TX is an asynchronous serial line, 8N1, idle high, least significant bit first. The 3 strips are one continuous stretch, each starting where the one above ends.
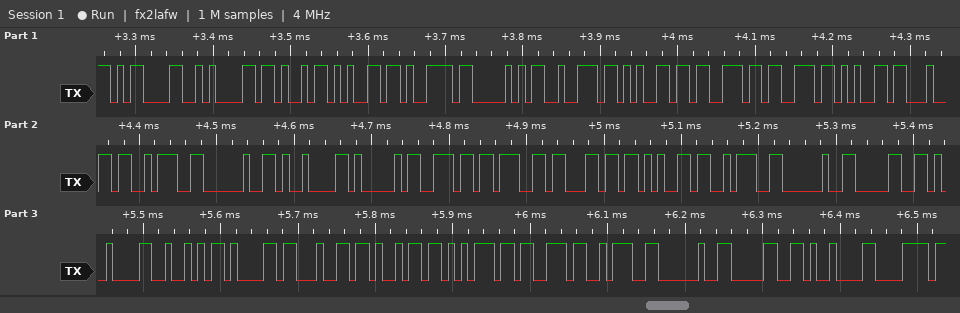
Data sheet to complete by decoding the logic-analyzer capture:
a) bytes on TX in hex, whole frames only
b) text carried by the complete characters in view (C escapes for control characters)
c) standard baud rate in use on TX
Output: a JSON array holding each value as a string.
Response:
["0D 0A 4B 65 79 50 72 65 73 73 65 64 3A 20 09 41 6E 67 6C 65 3A 20 30 09 52 61 64 69 75 73 3A 20 30 09 78", "\"\\r\\nKeyPressed: \\tAngle: 0\\tRadius: 0\\tx\"", "115200 baud"]
